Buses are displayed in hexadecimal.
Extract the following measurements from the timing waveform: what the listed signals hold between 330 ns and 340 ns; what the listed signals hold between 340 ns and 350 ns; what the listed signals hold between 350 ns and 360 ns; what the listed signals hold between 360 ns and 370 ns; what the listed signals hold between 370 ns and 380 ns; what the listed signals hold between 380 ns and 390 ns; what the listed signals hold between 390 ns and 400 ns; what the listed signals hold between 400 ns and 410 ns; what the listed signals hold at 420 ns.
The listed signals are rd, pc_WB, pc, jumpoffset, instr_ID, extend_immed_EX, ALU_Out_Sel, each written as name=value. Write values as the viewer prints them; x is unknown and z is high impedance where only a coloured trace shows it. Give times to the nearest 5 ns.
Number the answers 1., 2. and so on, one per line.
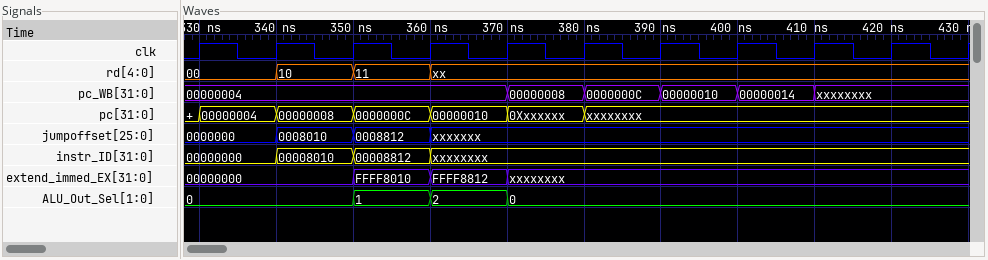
1. rd=00, pc_WB=00000004, pc=00000004, jumpoffset=0000000, instr_ID=00000000, extend_immed_EX=00000000, ALU_Out_Sel=0
2. rd=10, pc_WB=00000004, pc=00000008, jumpoffset=0008010, instr_ID=00008010, extend_immed_EX=00000000, ALU_Out_Sel=0
3. rd=11, pc_WB=00000004, pc=0000000C, jumpoffset=0008812, instr_ID=00008812, extend_immed_EX=FFFF8010, ALU_Out_Sel=1
4. rd=xx, pc_WB=00000004, pc=00000010, jumpoffset=xxxxxxx, instr_ID=xxxxxxxx, extend_immed_EX=FFFF8812, ALU_Out_Sel=2
5. rd=xx, pc_WB=00000008, pc=0Xxxxxxx, jumpoffset=xxxxxxx, instr_ID=xxxxxxxx, extend_immed_EX=xxxxxxxx, ALU_Out_Sel=0
6. rd=xx, pc_WB=0000000C, pc=xxxxxxxx, jumpoffset=xxxxxxx, instr_ID=xxxxxxxx, extend_immed_EX=xxxxxxxx, ALU_Out_Sel=0
7. rd=xx, pc_WB=00000010, pc=xxxxxxxx, jumpoffset=xxxxxxx, instr_ID=xxxxxxxx, extend_immed_EX=xxxxxxxx, ALU_Out_Sel=0
8. rd=xx, pc_WB=00000014, pc=xxxxxxxx, jumpoffset=xxxxxxx, instr_ID=xxxxxxxx, extend_immed_EX=xxxxxxxx, ALU_Out_Sel=0
9. rd=xx, pc_WB=xxxxxxxx, pc=xxxxxxxx, jumpoffset=xxxxxxx, instr_ID=xxxxxxxx, extend_immed_EX=xxxxxxxx, ALU_Out_Sel=0
